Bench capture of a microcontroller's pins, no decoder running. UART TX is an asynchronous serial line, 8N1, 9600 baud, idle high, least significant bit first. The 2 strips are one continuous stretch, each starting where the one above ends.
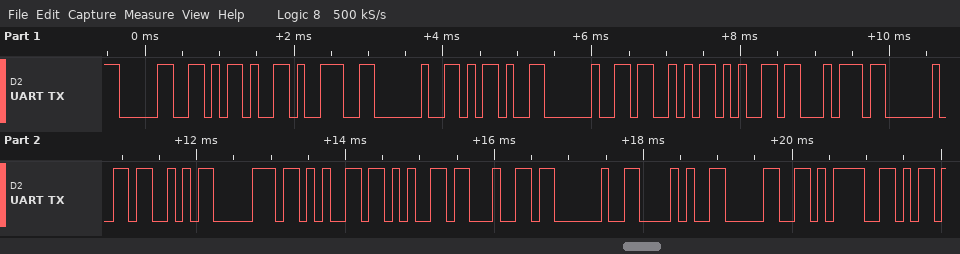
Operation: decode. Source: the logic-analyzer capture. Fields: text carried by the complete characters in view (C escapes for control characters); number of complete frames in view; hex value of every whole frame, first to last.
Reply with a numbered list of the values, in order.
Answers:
1. "0-9 - Set Speed (0="
2. 19
3. 30 2D 39 20 2D 20 53 65 74 20 53 70 65 65 64 20 28 30 3D
